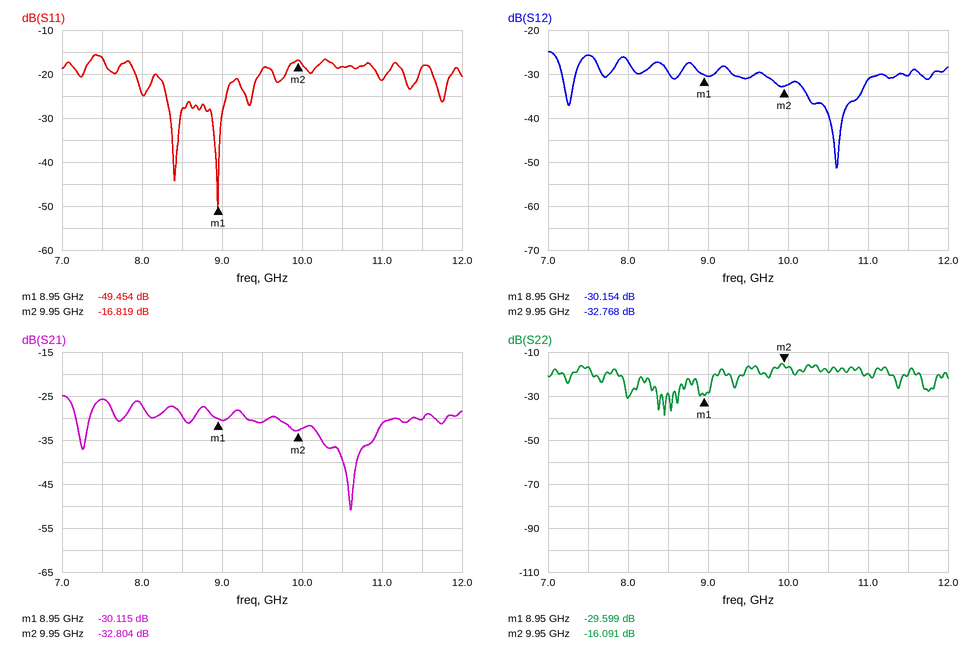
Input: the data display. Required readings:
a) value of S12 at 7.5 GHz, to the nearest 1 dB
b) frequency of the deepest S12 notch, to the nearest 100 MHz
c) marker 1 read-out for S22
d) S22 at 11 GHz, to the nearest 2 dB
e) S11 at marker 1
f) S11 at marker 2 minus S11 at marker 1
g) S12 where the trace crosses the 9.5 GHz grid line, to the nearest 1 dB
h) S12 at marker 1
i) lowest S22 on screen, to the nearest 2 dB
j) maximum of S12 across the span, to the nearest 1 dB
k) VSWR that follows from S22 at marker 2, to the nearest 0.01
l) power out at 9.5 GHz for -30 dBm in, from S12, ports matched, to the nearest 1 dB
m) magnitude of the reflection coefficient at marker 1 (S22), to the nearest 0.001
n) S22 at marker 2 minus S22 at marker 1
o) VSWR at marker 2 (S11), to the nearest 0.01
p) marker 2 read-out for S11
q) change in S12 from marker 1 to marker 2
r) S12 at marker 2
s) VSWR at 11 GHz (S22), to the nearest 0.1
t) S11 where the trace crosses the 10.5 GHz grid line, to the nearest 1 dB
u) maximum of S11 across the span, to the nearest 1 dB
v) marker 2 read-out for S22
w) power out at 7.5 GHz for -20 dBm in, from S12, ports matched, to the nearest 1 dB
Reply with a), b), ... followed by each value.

a) -26 dB
b) 10.6 GHz
c) -29.599 dB
d) -20 dB
e) -49.454 dB
f) 32.635 dB
g) -31 dB
h) -30.154 dB
i) -38 dB
j) -25 dB
k) 1.37
l) -61 dBm
m) 0.033
n) 13.508 dB
o) 1.34
p) -16.819 dB
q) -2.614 dB
r) -32.768 dB
s) 1.2
t) -18 dB
u) -16 dB
v) -16.091 dB
w) -46 dBm
